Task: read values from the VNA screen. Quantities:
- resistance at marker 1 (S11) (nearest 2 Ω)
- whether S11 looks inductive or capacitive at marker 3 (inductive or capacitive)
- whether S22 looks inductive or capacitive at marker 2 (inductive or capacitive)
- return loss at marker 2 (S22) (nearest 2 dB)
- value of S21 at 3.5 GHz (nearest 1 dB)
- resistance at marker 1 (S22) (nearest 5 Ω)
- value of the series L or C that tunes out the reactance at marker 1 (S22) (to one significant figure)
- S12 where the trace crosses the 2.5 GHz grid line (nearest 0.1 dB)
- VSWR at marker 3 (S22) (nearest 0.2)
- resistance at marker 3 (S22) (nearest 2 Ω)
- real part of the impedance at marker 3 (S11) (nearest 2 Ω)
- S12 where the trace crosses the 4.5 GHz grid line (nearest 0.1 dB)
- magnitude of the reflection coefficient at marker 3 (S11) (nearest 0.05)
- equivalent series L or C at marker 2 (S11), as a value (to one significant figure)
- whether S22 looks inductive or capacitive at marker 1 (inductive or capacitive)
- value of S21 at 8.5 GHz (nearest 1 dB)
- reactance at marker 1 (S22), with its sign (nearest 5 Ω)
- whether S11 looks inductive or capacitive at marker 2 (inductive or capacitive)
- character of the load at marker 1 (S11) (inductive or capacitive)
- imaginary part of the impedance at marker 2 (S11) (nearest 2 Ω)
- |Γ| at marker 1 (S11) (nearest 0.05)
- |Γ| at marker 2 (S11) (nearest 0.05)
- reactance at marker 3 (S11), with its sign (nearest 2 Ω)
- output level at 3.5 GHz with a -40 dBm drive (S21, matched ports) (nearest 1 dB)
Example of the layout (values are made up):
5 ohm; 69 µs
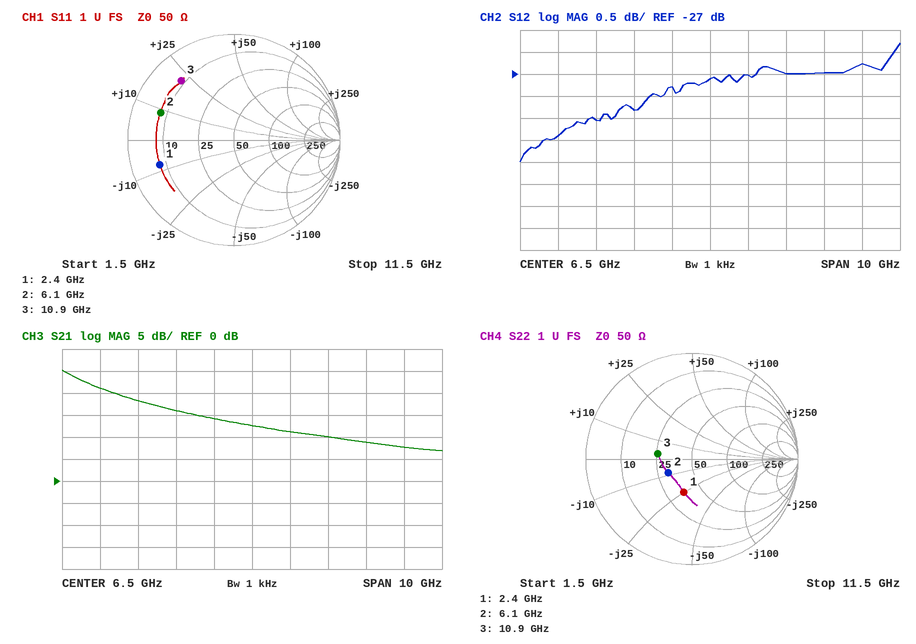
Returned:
8 Ω; inductive; capacitive; 12 dB; 18 dB; 35 Ω; 2 nH; -28.4 dB; 2.0; 26 Ω; 8 Ω; -27.8 dB; 0.75; 200 pH; capacitive; 10 dB; -25 Ω; inductive; capacitive; +8 Ω; 0.75; 0.75; +22 Ω; -22 dBm
